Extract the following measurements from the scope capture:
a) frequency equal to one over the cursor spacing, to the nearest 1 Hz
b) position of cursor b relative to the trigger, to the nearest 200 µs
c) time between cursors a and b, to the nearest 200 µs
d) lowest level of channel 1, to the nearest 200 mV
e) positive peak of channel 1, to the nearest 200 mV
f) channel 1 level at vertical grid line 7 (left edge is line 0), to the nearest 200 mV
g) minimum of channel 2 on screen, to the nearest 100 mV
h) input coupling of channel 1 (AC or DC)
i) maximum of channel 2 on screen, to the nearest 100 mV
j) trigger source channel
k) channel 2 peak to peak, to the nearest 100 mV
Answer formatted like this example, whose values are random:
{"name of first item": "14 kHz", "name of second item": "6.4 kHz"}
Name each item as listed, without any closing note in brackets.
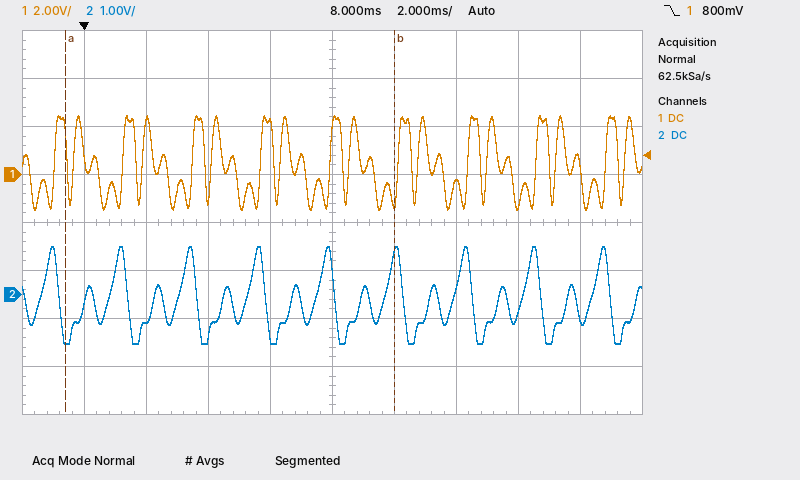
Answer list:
{"frequency equal to one over the cursor spacing, to the nearest 1 Hz": "94 Hz", "position of cursor b relative to the trigger, to the nearest 200 µs": "+10.0 ms", "time between cursors a and b, to the nearest 200 µs": "10.6 ms", "lowest level of channel 1, to the nearest 200 mV": "-1.4 V", "positive peak of channel 1, to the nearest 200 mV": "2.4 V", "channel 1 level at vertical grid line 7 (left edge is line 0), to the nearest 200 mV": "-400 mV", "minimum of channel 2 on screen, to the nearest 100 mV": "-1.0 V", "input coupling of channel 1": "DC", "maximum of channel 2 on screen, to the nearest 100 mV": "1.0 V", "trigger source channel": "channel 1", "channel 2 peak to peak, to the nearest 100 mV": "2.0 V"}
